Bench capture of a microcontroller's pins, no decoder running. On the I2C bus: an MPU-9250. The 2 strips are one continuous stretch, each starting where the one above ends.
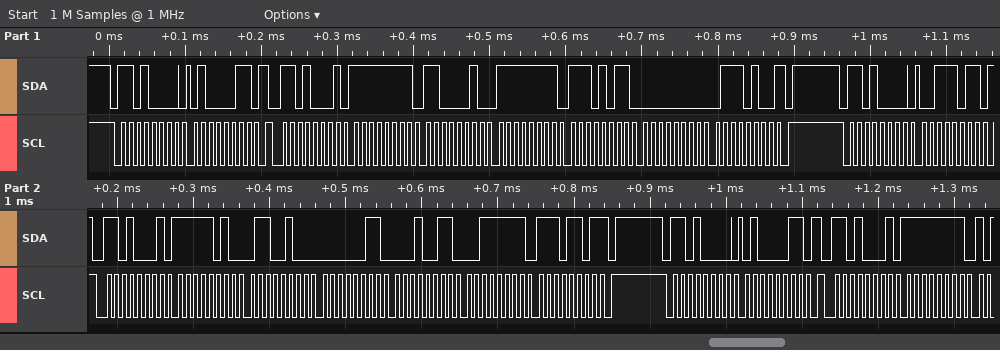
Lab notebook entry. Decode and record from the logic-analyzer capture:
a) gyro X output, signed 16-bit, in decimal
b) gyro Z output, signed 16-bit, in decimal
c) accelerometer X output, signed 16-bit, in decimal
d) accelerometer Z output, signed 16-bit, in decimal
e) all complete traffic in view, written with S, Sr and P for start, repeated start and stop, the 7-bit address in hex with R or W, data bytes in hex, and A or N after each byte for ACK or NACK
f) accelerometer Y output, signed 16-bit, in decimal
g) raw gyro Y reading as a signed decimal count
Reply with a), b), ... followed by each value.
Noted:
a) -62
b) 116
c) -1436
d) 16365
e) S 68W A 43 A Sr 68R A FF A C2 A FF A EB A 00 A 74 N P S 68W A 3B A Sr 68R A FA A 64 A 03 A 13 A 3F A ED N P S 68W A 43 A Sr 68R A FF A
f) 787
g) -21
